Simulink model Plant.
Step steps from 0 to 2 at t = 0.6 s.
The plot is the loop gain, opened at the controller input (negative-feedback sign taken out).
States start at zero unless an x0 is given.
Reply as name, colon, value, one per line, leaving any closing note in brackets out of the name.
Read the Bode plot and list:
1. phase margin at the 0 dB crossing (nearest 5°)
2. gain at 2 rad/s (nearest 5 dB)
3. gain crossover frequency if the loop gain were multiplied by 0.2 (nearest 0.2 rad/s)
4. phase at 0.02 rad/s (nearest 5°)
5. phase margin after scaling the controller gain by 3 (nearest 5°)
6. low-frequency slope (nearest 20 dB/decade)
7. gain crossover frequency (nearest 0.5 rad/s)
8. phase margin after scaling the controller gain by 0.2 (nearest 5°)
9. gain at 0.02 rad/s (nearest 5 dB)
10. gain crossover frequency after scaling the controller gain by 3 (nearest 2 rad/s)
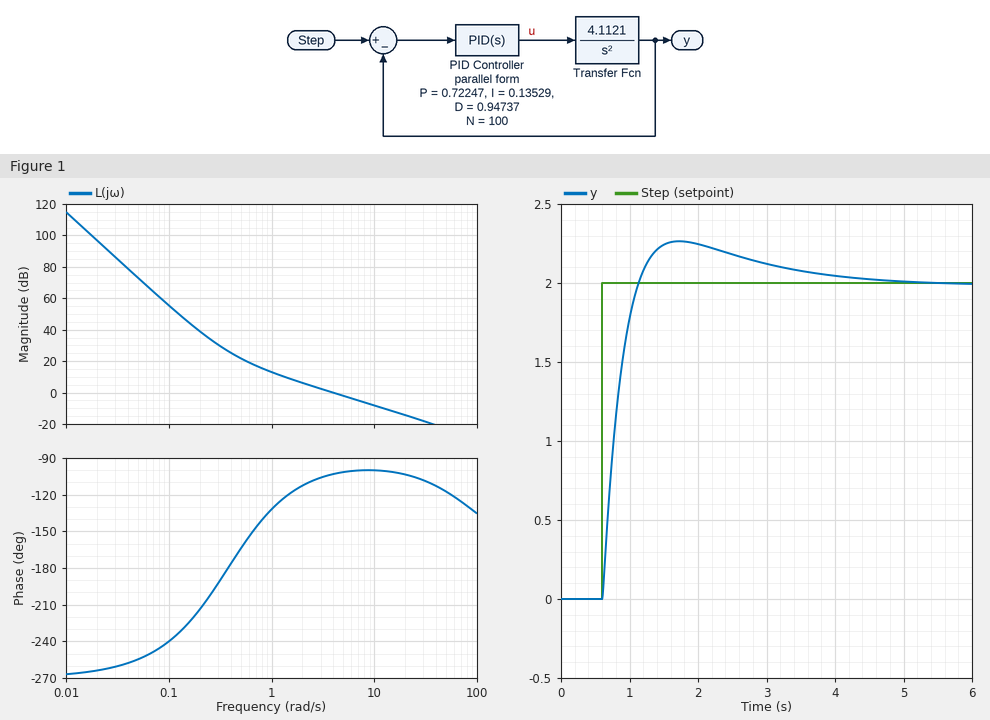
phase margin at the 0 dB crossing: 75°
gain at 2 rad/s: 5 dB
gain crossover frequency if the loop gain were multiplied by 0.2: 1.0 rad/s
phase at 0.02 rad/s: -265°
phase margin after scaling the controller gain by 3: 80°
low-frequency slope: -60 dB/decade
gain crossover frequency: 4.0 rad/s
phase margin after scaling the controller gain by 0.2: 45°
gain at 0.02 rad/s: 95 dB
gain crossover frequency after scaling the controller gain by 3: 12 rad/s
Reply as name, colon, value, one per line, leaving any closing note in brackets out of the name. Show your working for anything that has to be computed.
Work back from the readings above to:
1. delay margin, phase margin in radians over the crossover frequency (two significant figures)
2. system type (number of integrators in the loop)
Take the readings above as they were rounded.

delay margin, phase margin in radians over the crossover frequency: 75 × π / 180 / 4 = 0.33 s
system type: 3
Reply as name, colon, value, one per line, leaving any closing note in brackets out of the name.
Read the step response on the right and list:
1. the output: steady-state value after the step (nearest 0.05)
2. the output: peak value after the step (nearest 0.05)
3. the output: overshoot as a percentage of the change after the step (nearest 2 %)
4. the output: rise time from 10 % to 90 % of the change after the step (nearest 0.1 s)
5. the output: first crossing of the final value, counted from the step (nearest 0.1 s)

the output: steady-state value after the step: 2.00
the output: peak value after the step: 2.25
the output: overshoot as a percentage of the change after the step: 14 %
the output: rise time from 10 % to 90 % of the change after the step: 0.4 s
the output: first crossing of the final value, counted from the step: 0.5 s
